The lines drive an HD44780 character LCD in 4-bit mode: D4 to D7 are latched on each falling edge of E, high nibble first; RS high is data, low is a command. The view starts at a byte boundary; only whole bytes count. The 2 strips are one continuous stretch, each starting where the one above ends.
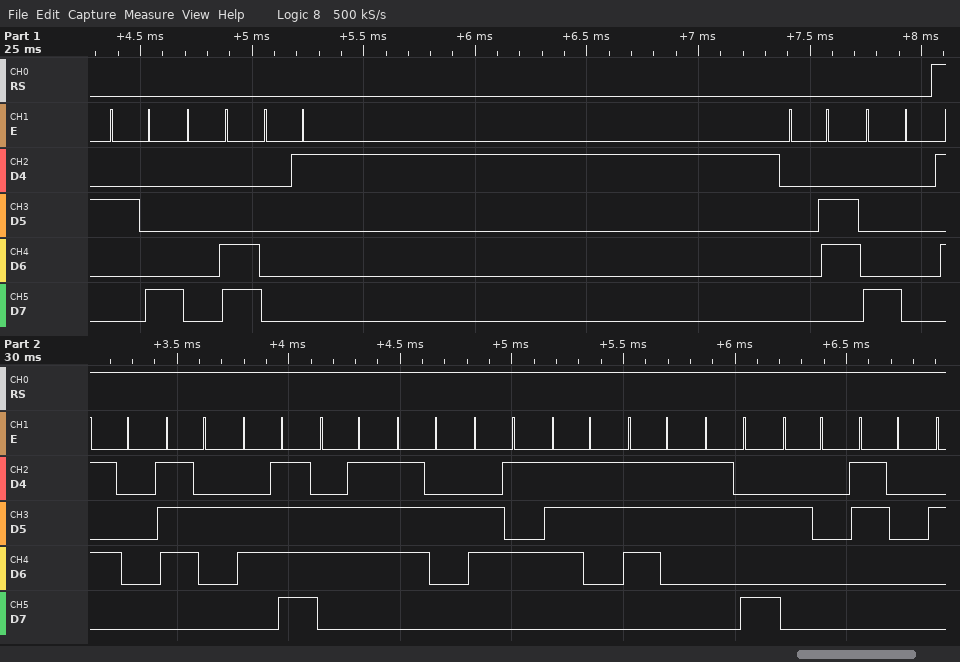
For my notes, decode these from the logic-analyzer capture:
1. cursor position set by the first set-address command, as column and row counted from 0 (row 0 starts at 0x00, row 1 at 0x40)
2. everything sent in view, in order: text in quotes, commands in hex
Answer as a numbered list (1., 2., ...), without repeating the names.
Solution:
1. column 0, row 0
2. 0x28 0x0C 0x01 0x06 0x80 "Progress: 0"
